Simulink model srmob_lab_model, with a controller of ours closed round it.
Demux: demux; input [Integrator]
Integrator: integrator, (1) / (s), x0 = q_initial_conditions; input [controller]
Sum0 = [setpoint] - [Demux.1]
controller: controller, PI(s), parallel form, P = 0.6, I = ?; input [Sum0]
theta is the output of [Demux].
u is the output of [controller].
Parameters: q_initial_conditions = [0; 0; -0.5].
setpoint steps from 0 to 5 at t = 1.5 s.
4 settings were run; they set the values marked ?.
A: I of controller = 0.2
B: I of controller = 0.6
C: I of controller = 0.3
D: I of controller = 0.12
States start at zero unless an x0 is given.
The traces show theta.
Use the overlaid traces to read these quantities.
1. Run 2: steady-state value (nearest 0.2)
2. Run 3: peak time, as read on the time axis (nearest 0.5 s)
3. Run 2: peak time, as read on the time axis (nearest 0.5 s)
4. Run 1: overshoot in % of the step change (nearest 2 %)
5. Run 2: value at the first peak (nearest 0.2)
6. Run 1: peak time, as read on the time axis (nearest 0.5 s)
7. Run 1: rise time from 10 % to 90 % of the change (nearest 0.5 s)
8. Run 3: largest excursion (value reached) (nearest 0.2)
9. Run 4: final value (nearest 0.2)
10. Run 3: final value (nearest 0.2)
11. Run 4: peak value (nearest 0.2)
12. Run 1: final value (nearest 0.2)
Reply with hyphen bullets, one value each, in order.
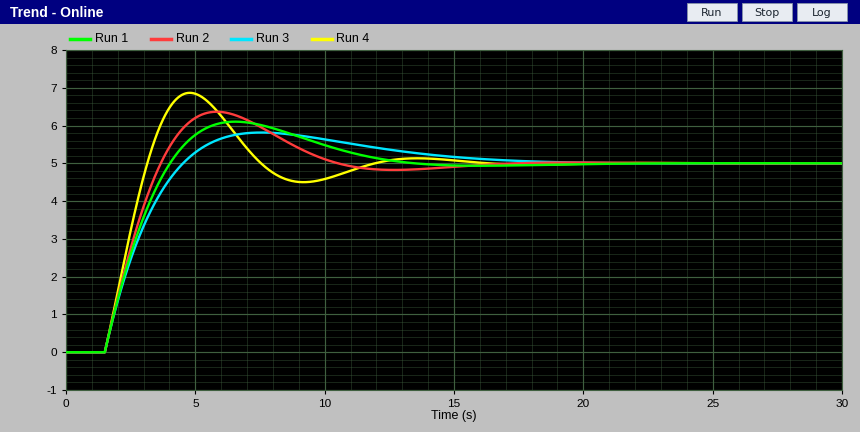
- 5.0
- 7.5 s
- 6.0 s
- 22 %
- 6.4
- 6.5 s
- 2.0 s
- 5.8
- 5.0
- 5.0
- 6.8
- 5.0
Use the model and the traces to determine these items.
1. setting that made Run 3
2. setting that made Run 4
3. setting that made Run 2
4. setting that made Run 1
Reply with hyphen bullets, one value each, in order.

- D
- B
- C
- A
